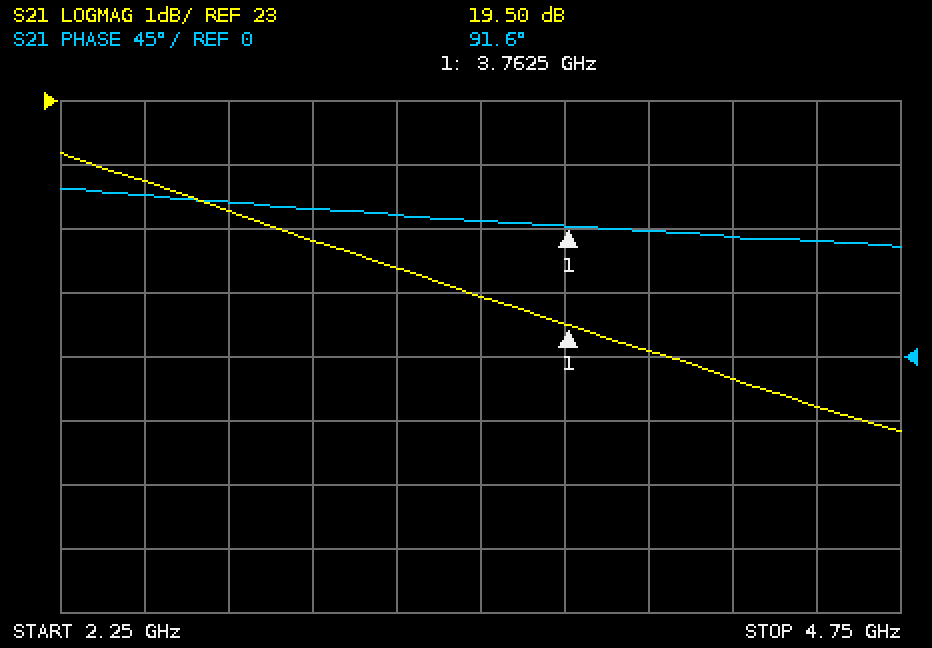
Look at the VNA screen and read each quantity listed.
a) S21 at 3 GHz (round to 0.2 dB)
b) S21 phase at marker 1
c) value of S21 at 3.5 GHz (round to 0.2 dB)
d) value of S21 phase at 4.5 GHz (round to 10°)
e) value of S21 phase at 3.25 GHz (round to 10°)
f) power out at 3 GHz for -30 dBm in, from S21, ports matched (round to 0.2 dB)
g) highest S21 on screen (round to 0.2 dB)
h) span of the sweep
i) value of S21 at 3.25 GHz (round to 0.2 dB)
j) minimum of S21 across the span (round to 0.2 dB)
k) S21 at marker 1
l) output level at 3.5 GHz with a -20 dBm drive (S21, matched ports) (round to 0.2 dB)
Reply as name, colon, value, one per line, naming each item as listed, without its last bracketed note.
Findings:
S21 at 3 GHz: 20.8 dB
S21 phase at marker 1: 91.6°
value of S21 at 3.5 GHz: 20.0 dB
value of S21 phase at 4.5 GHz: 80°
value of S21 phase at 3.25 GHz: 100°
power out at 3 GHz for -30 dBm in, from S21, ports matched: -9.2 dBm
highest S21 on screen: 22.2 dB
span of the sweep: 2.5 GHz
value of S21 at 3.25 GHz: 20.4 dB
minimum of S21 across the span: 17.8 dB
S21 at marker 1: 19.50 dB
output level at 3.5 GHz with a -20 dBm drive (S21, matched ports): 0.0 dBm
